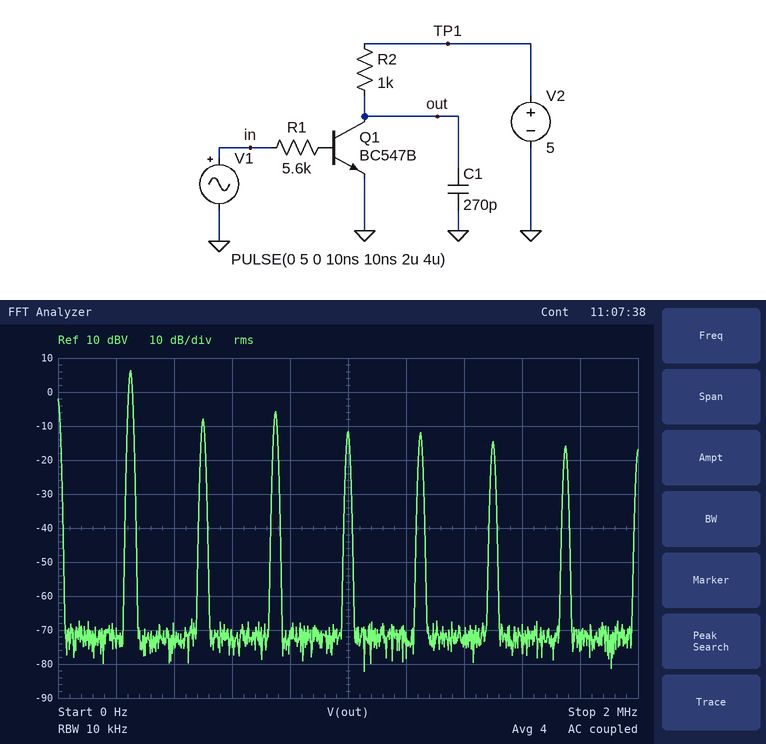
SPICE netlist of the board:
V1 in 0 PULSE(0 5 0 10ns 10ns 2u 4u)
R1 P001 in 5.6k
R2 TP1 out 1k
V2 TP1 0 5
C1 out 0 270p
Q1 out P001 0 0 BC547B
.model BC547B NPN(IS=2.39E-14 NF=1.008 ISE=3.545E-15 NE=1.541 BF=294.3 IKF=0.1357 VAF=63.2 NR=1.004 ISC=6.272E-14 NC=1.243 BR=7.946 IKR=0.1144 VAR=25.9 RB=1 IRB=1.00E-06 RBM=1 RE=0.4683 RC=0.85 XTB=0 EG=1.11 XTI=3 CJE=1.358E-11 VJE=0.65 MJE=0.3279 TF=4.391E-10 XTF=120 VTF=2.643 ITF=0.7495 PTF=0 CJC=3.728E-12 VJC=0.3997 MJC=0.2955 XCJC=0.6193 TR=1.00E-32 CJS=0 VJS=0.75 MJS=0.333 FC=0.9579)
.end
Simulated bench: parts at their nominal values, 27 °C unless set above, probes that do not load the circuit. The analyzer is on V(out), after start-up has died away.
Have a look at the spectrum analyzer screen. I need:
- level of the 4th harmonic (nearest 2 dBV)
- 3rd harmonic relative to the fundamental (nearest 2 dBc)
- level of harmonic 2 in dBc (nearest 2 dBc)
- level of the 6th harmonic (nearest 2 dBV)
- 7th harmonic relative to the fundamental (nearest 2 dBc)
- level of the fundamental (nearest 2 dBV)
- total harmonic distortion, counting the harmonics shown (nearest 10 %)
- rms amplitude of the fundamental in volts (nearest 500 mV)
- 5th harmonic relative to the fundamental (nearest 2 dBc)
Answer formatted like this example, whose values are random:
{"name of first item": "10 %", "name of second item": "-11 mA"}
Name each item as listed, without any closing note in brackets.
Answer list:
{"level of the 4th harmonic": "-12 dBV", "3rd harmonic relative to the fundamental": "-12 dBc", "level of harmonic 2 in dBc": "-14 dBc", "level of the 6th harmonic": "-14 dBV", "7th harmonic relative to the fundamental": "-22 dBc", "level of the fundamental": "6 dBV", "total harmonic distortion, counting the harmonics shown": "40 %", "rms amplitude of the fundamental in volts": "2.0 V", "5th harmonic relative to the fundamental": "-18 dBc"}
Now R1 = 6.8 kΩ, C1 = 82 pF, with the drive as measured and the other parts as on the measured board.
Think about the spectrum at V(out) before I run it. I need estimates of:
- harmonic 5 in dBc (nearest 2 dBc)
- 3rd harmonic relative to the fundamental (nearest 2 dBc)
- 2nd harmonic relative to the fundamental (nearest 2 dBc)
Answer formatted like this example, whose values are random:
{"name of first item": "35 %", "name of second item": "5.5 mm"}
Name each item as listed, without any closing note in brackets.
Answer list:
{"harmonic 5 in dBc": "-16 dBc", "3rd harmonic relative to the fundamental": "-10 dBc", "2nd harmonic relative to the fundamental": "-18 dBc"}
